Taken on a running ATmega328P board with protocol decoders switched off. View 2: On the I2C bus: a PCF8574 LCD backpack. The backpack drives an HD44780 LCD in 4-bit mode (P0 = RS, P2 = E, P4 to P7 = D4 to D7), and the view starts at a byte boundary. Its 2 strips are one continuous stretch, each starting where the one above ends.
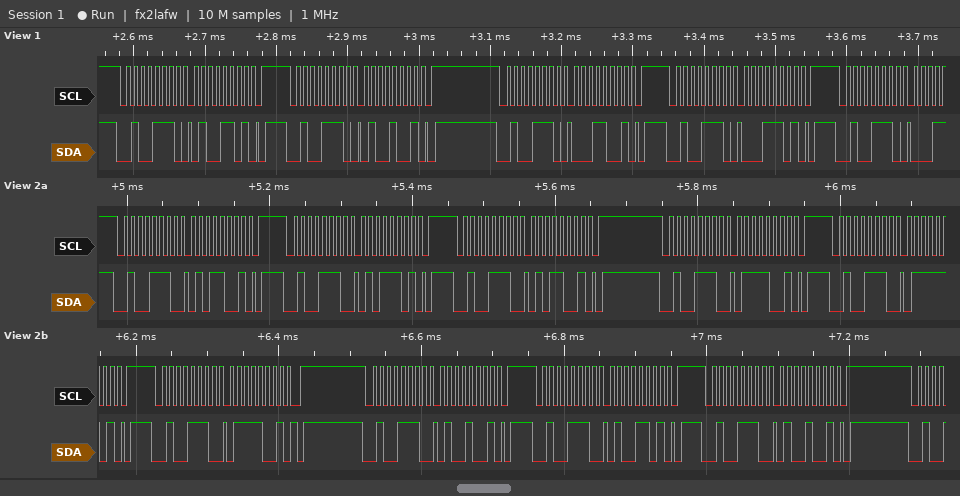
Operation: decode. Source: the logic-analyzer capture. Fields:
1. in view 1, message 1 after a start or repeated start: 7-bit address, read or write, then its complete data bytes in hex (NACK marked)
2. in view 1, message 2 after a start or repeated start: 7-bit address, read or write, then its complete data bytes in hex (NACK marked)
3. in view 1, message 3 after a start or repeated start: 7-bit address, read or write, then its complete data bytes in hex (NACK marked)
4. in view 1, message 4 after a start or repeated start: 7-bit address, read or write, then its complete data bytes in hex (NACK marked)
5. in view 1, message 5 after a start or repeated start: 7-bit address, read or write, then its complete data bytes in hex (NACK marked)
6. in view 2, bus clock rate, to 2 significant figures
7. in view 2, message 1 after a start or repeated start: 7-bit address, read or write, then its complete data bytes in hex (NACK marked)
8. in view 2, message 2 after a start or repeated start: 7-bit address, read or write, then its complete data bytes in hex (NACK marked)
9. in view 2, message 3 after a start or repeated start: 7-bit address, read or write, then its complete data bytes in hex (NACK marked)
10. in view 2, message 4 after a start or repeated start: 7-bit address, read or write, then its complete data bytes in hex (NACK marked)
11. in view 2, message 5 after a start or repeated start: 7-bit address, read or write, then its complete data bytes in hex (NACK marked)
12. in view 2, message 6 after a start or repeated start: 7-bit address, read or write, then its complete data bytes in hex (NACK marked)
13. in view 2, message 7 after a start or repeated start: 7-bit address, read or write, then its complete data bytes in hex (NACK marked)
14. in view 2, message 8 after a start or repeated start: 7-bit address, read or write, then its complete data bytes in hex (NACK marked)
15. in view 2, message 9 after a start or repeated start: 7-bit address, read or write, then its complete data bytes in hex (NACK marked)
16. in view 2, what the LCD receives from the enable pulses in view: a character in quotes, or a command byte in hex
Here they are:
0x27 write: 4D
0x27 write: 49
0x27 write: 19
0x27 write: 1D
0x27 write
100 kHz
0x27 write: 59
0x27 write: 5D
0x27 write: 59
0x27 write: 79
0x27 write: 7D
0x27 write: 79
0x27 write: 49
0x27 write: 4D
0x27 write: 49
'W'
